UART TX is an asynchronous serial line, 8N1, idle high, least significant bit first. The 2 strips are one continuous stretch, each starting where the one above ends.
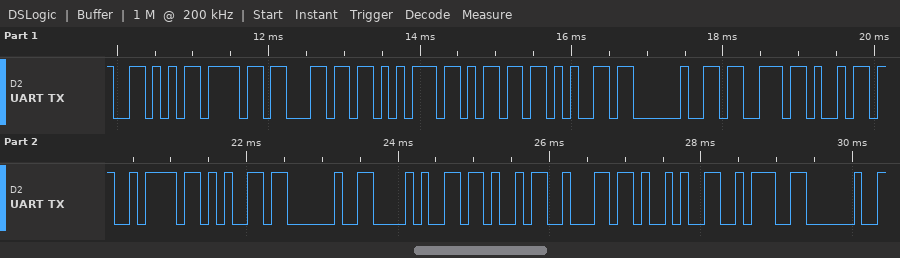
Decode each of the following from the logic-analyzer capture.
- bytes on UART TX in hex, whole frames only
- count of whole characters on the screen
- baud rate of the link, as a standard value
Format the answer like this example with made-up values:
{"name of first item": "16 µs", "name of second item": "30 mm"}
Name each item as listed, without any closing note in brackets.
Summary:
{"bytes on UART TX in hex, whole frames only": "0x56 0x6F 0x6C 0x75 0x6D 0x65 0x20 0x73 0x69 0x7A 0x65 0x20 0x28 0x4B 0x62 0x29 0x3A 0x20", "count of whole characters on the screen": "18", "baud rate of the link, as a standard value": "9600 baud"}
